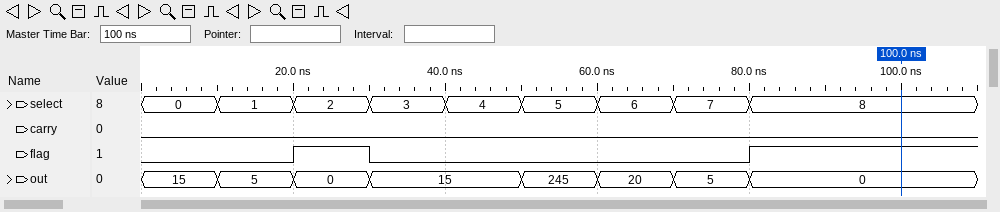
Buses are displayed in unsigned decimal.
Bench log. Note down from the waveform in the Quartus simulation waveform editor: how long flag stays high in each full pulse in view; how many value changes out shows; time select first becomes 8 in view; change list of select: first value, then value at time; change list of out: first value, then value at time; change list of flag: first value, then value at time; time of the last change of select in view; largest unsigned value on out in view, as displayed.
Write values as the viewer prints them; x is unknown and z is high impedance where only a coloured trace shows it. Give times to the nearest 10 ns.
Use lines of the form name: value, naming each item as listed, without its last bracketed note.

how long flag stays high in each full pulse in view: 10 ns
how many value changes out shows: 7
time select first becomes 8 in view: 80 ns
change list of select: first value, then value at time: 0, 1 at 10 ns, 2 at 20 ns, 3 at 30 ns, 4 at 40 ns, 5 at 50 ns, 6 at 60 ns, 7 at 70 ns, 8 at 80 ns
change list of out: first value, then value at time: 15, 5 at 10 ns, 0 at 20 ns, 15 at 30 ns, 245 at 50 ns, 20 at 60 ns, 5 at 70 ns, 0 at 80 ns
change list of flag: first value, then value at time: 0, 1 at 20 ns, 0 at 30 ns, 1 at 80 ns
time of the last change of select in view: 80 ns
largest unsigned value on out in view, as displayed: 245
